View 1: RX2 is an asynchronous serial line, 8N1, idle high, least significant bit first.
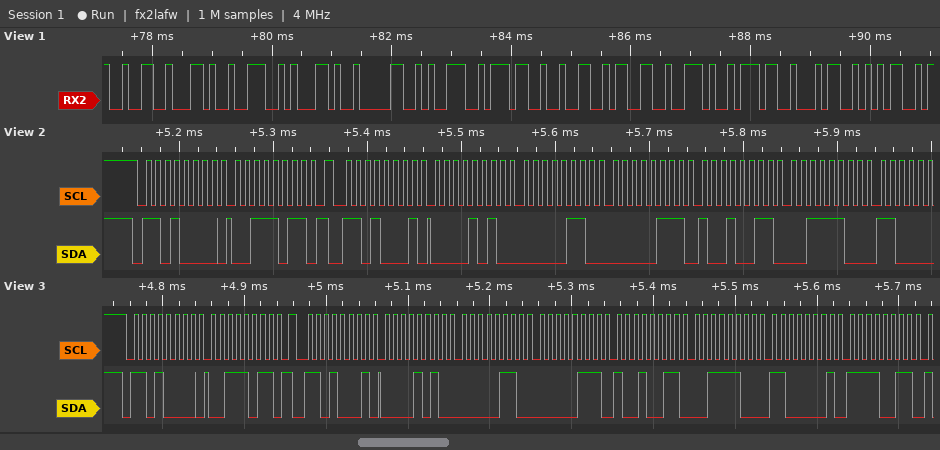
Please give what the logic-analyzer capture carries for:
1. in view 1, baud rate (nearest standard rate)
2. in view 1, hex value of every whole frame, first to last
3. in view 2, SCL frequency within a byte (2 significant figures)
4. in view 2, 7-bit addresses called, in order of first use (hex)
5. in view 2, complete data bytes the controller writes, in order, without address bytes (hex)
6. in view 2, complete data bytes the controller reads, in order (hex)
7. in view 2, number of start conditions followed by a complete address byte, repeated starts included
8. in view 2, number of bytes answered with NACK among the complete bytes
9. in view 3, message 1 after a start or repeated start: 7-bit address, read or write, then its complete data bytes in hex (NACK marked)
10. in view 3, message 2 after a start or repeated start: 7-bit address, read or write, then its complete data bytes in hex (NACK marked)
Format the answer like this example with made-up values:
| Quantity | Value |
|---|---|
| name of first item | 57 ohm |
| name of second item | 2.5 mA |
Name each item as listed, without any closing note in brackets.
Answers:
| Quantity | Value |
|---|---|
| in view 1, baud rate | 9600 baud |
| in view 1, hex value of every whole frame, first to last | 32 2C 4E 2C 30 39 37 32 33 2E 37 34 35 |
| in view 2, SCL frequency within a byte | 100 kHz |
| in view 2, 7-bit addresses called, in order of first use | 0x68 |
| in view 2, complete data bytes the controller writes, in order, without address bytes | 3B |
| in view 2, complete data bytes the controller reads, in order | 0A 06 07 93 3C |
| in view 2, number of start conditions followed by a complete address byte, repeated starts included | 2 |
| in view 2, number of bytes answered with NACK among the complete bytes | 0 |
| in view 3, message 1 after a start or repeated start: 7-bit address, read or write, then its complete data bytes in hex | 0x68 write: 3B |
| in view 3, message 2 after a start or repeated start: 7-bit address, read or write, then its complete data bytes in hex | 0x68 read: 0A 06 07 93 3C C1 F3 |
